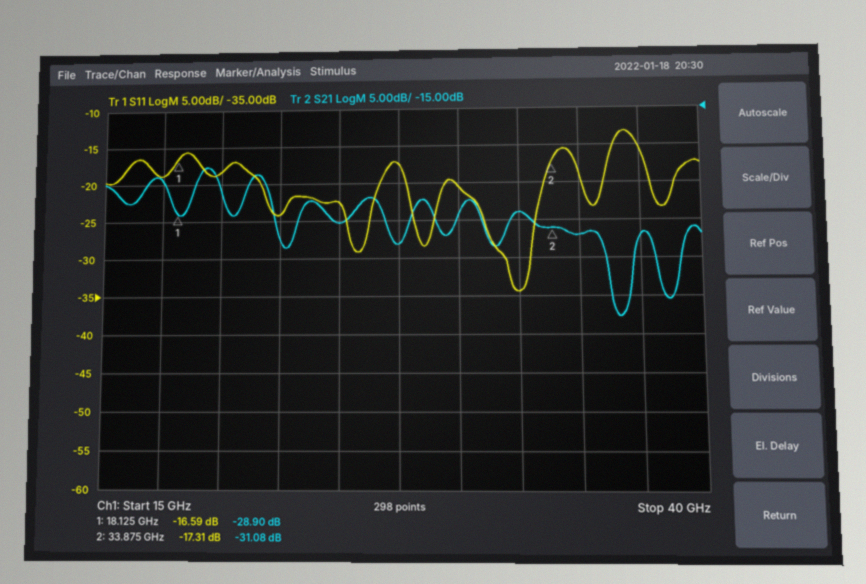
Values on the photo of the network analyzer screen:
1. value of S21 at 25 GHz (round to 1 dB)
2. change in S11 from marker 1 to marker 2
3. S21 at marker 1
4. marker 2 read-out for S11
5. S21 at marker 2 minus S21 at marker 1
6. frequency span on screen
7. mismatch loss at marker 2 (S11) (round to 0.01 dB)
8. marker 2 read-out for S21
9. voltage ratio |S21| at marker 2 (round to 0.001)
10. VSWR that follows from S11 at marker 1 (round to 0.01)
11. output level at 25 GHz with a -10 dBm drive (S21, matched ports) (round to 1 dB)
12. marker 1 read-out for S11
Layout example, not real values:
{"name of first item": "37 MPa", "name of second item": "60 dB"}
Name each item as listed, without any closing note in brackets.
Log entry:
{"value of S21 at 25 GHz": "-30 dB", "change in S11 from marker 1 to marker 2": "-0.72 dB", "S21 at marker 1": "-28.90 dB", "marker 2 read-out for S11": "-17.31 dB", "S21 at marker 2 minus S21 at marker 1": "-2.18 dB", "frequency span on screen": "25 GHz", "mismatch loss at marker 2 (S11)": "0.08 dB", "marker 2 read-out for S21": "-31.08 dB", "voltage ratio |S21| at marker 2": "0.028", "VSWR that follows from S11 at marker 1": "1.35", "output level at 25 GHz with a -10 dBm drive (S21, matched ports)": "-40 dBm", "marker 1 read-out for S11": "-16.59 dB"}
